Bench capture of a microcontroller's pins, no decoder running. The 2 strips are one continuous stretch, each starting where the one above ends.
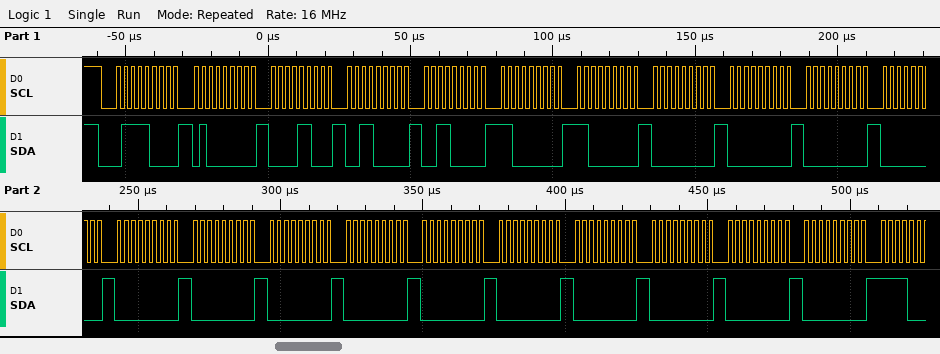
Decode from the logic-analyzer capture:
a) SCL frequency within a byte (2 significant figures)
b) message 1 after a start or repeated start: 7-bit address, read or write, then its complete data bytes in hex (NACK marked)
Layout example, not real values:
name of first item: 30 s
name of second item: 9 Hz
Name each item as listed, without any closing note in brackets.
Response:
SCL frequency within a byte: 400 kHz
message 1 after a start or repeated start: 7-bit address, read or write, then its complete data bytes in hex: 0x3C write: 40 0C 30 30 C0 C0 00 00 00 00 00 00 00 00 00 00 00 00 00 00
